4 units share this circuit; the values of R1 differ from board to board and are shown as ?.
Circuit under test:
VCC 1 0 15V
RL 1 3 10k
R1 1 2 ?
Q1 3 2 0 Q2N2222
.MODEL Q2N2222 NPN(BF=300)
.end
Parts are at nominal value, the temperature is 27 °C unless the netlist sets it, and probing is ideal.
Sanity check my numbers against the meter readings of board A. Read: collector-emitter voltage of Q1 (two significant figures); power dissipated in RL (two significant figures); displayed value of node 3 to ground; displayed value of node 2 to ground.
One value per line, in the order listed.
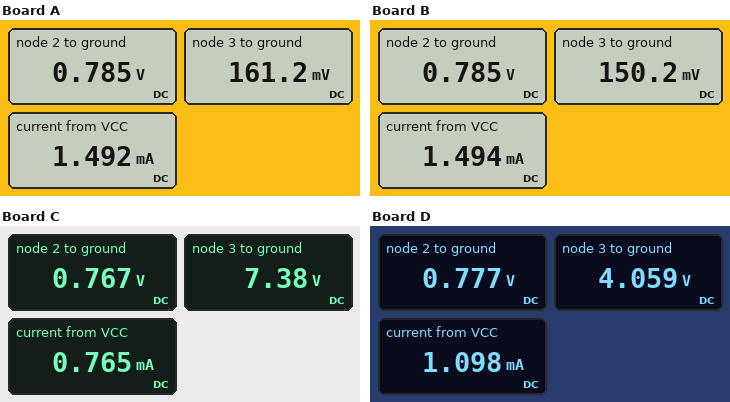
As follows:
160 mV
22 mW
161.2 mV
0.785 V
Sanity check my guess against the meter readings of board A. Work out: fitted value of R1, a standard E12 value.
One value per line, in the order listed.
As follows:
1.8 MΩ
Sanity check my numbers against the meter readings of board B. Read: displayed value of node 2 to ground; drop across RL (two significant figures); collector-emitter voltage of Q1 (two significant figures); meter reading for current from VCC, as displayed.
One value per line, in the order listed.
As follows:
0.785 V
15 V
150 mV
1.494 mA
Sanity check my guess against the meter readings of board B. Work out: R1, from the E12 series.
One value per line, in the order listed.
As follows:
1.5 MΩ
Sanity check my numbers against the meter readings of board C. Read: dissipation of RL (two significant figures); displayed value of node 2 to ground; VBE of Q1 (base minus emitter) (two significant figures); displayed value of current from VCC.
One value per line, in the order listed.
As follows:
5.8 mW
0.767 V
770 mV
0.765 mA
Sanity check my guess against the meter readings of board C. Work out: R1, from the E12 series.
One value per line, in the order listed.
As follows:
5.6 MΩ
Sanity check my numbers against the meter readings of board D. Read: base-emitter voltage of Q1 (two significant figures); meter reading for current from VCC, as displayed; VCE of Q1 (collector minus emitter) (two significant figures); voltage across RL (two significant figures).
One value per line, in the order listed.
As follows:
780 mV
1.098 mA
4.1 V
11 V
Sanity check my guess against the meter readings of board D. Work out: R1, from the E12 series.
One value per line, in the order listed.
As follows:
3.9 MΩ
